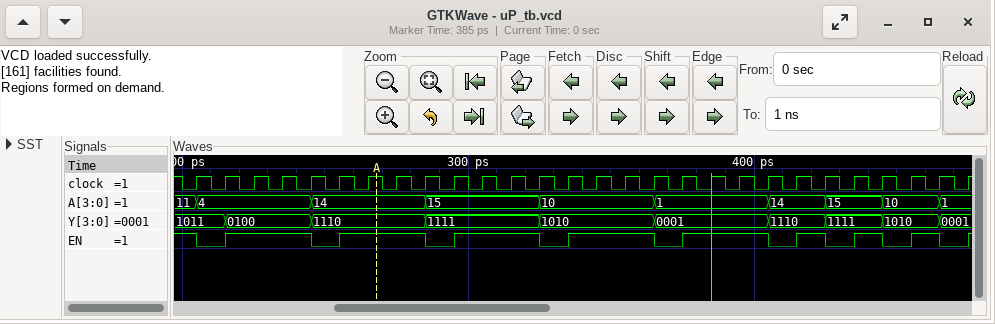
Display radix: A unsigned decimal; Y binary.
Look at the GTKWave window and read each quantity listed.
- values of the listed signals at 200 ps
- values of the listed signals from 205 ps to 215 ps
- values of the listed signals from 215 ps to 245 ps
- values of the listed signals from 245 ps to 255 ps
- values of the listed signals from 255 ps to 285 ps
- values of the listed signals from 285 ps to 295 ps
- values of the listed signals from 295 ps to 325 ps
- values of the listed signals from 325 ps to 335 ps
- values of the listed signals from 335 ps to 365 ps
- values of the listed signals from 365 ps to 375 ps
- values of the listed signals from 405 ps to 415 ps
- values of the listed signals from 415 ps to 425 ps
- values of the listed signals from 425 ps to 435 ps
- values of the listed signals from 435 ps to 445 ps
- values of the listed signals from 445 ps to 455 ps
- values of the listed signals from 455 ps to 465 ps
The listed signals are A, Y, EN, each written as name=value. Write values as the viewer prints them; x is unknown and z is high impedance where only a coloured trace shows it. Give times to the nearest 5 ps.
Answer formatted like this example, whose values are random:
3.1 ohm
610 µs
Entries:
A=11, Y=1011, EN=1
A=4, Y=1011, EN=0
A=4, Y=0100, EN=1
A=14, Y=1110, EN=0
A=14, Y=1110, EN=1
A=15, Y=1111, EN=0
A=15, Y=1111, EN=1
A=10, Y=1010, EN=0
A=10, Y=1010, EN=1
A=1, Y=0001, EN=0
A=14, Y=1110, EN=0
A=14, Y=1110, EN=1
A=15, Y=1111, EN=0
A=15, Y=1111, EN=1
A=10, Y=1010, EN=0
A=10, Y=1010, EN=1
